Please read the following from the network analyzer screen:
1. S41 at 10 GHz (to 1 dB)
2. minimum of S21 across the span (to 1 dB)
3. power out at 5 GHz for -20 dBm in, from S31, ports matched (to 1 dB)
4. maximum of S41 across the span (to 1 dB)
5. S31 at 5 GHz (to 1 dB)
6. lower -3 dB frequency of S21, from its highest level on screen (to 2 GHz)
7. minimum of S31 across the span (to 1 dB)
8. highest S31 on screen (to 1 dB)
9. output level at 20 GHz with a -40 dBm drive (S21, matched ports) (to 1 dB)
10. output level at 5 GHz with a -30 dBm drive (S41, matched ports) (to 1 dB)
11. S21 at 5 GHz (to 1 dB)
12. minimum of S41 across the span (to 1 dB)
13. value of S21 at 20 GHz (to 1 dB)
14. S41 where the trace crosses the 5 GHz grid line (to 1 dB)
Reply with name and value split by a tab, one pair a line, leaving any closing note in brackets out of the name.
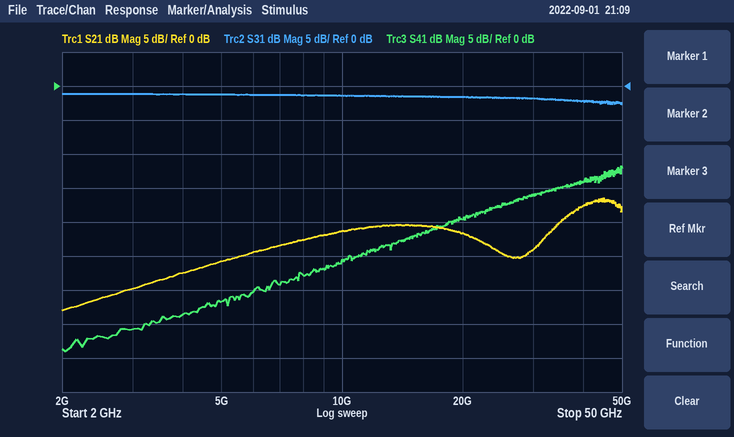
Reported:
S41 at 10 GHz	-26 dB
minimum of S21 across the span	-33 dB
power out at 5 GHz for -20 dBm in, from S31, ports matched	-21 dBm
maximum of S41 across the span	-12 dB
S31 at 5 GHz	-1 dB
lower -3 dB frequency of S21, from its highest level on screen	36 GHz
minimum of S31 across the span	-3 dB
highest S31 on screen	-1 dB
output level at 20 GHz with a -40 dBm drive (S21, matched ports)	-62 dBm
output level at 5 GHz with a -30 dBm drive (S41, matched ports)	-62 dBm
S21 at 5 GHz	-26 dB
minimum of S41 across the span	-39 dB
value of S21 at 20 GHz	-22 dB
S41 where the trace crosses the 5 GHz grid line	-32 dB
